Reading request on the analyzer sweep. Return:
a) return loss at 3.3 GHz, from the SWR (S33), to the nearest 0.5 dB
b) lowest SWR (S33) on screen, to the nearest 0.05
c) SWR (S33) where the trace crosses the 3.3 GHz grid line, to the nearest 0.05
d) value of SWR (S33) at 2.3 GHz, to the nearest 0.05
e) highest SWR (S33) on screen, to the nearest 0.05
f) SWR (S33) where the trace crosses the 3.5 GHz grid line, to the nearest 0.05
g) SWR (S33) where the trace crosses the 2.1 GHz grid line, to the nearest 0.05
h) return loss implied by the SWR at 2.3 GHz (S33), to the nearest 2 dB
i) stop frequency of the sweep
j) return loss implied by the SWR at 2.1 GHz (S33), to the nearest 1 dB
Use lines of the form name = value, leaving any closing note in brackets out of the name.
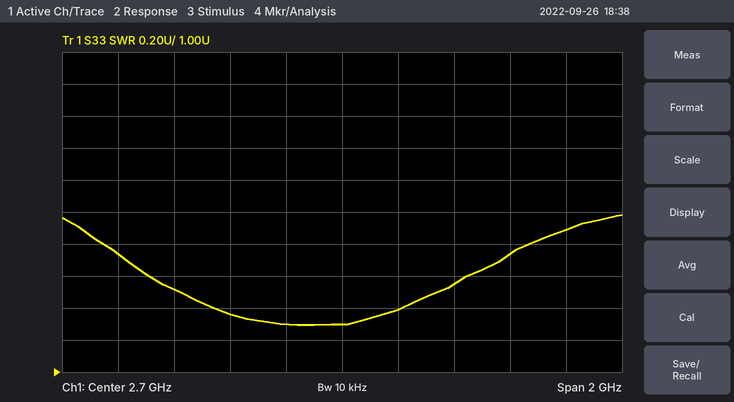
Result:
return loss at 3.3 GHz, from the SWR (S33), to the nearest 0.5 dB = 11.5 dB
lowest SWR (S33) on screen, to the nearest 0.05 = 1.30
SWR (S33) where the trace crosses the 3.3 GHz grid line, to the nearest 0.05 = 1.75
value of SWR (S33) at 2.3 GHz, to the nearest 0.05 = 1.35
highest SWR (S33) on screen, to the nearest 0.05 = 2.00
SWR (S33) where the trace crosses the 3.5 GHz grid line, to the nearest 0.05 = 1.90
SWR (S33) where the trace crosses the 2.1 GHz grid line, to the nearest 0.05 = 1.50
return loss implied by the SWR at 2.3 GHz (S33), to the nearest 2 dB = 16 dB
stop frequency of the sweep = 3.7 GHz
return loss implied by the SWR at 2.1 GHz (S33), to the nearest 1 dB = 14 dB
